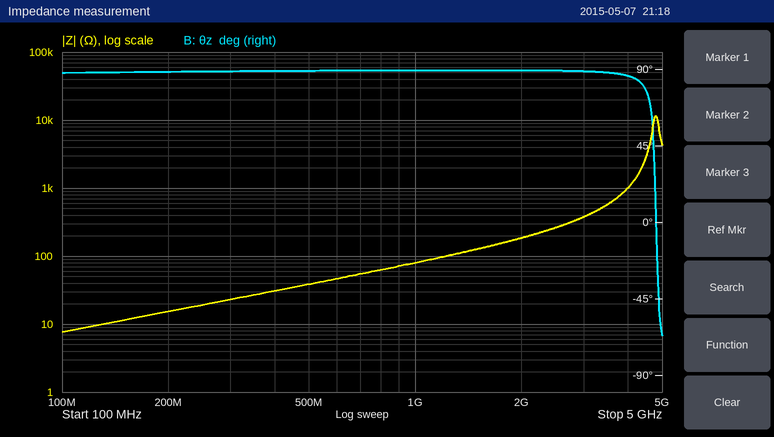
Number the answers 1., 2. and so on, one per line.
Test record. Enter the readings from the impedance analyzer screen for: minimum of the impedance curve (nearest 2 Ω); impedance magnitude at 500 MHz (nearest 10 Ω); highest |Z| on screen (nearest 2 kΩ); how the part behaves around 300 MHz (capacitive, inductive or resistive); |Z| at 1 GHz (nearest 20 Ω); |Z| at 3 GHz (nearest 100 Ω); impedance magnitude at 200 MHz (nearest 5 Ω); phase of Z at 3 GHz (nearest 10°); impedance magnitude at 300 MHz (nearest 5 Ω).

1. 8 Ω
2. 40 Ω
3. 12 kΩ
4. inductive
5. 80 Ω
6. 400 Ω
7. 15 Ω
8. 90°
9. 25 Ω
